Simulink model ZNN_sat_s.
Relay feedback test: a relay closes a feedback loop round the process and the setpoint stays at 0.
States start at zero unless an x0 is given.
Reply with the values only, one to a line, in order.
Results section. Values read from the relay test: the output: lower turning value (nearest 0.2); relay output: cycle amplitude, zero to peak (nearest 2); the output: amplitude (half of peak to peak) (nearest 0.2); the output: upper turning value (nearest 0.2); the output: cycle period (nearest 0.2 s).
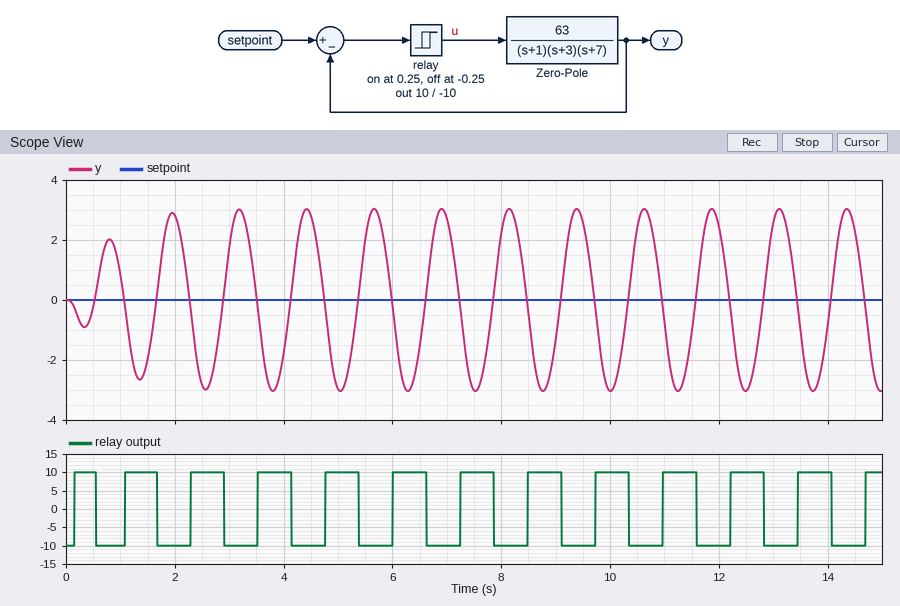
-3.0
10
3.0
3.0
1.2 s
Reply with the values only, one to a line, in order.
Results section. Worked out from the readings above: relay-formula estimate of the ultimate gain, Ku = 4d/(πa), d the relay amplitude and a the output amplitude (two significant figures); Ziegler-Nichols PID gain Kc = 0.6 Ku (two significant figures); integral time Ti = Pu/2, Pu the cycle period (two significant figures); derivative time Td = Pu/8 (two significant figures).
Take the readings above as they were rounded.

4.2
2.5
0.60 s
0.15 s
